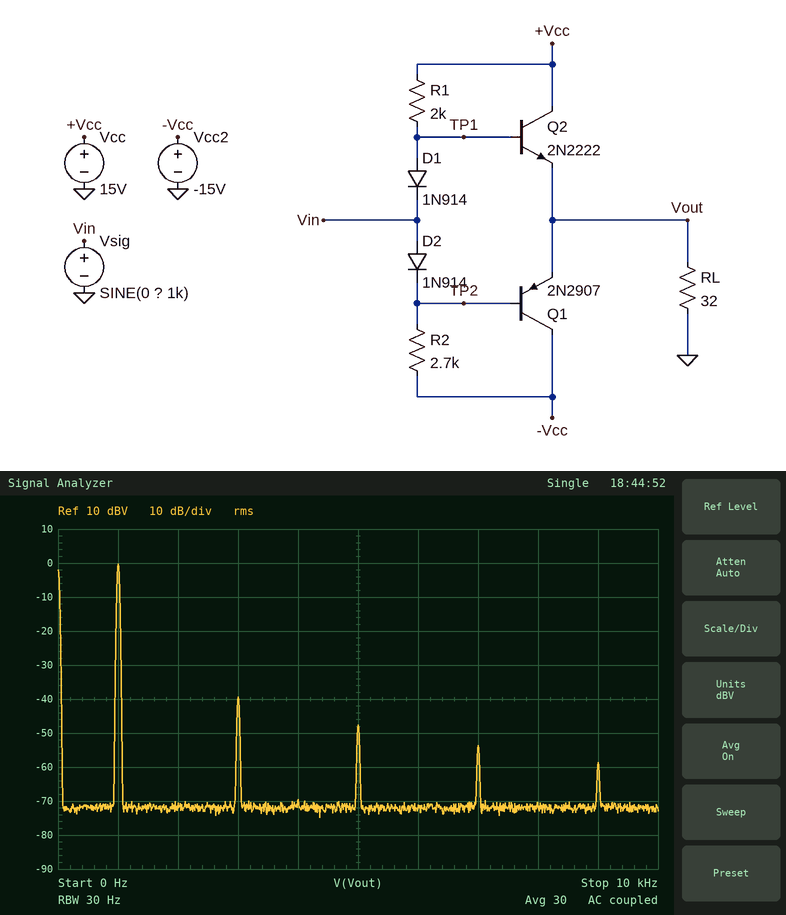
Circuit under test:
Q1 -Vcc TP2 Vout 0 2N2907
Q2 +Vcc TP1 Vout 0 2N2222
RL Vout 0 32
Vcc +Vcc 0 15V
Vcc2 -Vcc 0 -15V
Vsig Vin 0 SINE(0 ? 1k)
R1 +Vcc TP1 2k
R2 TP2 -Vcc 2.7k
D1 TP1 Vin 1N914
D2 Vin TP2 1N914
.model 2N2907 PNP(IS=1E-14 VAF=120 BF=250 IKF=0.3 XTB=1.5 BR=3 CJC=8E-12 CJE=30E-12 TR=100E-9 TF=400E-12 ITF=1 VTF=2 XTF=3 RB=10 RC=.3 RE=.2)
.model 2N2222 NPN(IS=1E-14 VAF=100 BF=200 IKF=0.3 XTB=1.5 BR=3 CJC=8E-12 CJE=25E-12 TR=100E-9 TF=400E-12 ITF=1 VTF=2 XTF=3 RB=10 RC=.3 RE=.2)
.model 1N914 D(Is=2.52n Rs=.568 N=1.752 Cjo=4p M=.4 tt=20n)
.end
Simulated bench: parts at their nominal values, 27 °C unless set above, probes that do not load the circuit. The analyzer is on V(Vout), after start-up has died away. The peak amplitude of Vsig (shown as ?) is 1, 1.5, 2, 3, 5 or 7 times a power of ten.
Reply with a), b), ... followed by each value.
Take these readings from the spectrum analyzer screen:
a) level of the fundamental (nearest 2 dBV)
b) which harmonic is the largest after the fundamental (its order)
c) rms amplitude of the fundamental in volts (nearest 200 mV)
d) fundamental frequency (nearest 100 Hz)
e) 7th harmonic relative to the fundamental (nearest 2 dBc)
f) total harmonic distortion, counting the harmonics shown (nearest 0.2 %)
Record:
a) 0 dBV
b) 3
c) 1.0 V
d) 1.0 kHz
e) -54 dBc
f) 1.2 %
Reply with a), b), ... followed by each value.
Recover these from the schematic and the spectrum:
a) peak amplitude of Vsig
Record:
a) 1.5 V
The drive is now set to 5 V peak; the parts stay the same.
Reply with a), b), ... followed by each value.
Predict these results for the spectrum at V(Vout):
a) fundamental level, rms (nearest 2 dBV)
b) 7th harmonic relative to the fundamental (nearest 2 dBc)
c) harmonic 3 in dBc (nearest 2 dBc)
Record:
a) 10 dBV
b) -56 dBc
c) -46 dBc
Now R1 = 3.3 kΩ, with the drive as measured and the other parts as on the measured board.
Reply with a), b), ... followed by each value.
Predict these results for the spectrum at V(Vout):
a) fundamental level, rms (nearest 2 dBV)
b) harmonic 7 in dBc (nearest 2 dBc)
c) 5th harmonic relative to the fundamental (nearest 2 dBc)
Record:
a) 0 dBV
b) -50 dBc
c) -44 dBc
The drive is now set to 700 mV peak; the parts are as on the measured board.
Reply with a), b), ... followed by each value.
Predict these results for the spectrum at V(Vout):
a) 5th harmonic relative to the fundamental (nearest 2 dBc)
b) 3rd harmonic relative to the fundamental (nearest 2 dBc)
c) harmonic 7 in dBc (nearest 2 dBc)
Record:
a) -48 dBc
b) -38 dBc
c) -58 dBc
